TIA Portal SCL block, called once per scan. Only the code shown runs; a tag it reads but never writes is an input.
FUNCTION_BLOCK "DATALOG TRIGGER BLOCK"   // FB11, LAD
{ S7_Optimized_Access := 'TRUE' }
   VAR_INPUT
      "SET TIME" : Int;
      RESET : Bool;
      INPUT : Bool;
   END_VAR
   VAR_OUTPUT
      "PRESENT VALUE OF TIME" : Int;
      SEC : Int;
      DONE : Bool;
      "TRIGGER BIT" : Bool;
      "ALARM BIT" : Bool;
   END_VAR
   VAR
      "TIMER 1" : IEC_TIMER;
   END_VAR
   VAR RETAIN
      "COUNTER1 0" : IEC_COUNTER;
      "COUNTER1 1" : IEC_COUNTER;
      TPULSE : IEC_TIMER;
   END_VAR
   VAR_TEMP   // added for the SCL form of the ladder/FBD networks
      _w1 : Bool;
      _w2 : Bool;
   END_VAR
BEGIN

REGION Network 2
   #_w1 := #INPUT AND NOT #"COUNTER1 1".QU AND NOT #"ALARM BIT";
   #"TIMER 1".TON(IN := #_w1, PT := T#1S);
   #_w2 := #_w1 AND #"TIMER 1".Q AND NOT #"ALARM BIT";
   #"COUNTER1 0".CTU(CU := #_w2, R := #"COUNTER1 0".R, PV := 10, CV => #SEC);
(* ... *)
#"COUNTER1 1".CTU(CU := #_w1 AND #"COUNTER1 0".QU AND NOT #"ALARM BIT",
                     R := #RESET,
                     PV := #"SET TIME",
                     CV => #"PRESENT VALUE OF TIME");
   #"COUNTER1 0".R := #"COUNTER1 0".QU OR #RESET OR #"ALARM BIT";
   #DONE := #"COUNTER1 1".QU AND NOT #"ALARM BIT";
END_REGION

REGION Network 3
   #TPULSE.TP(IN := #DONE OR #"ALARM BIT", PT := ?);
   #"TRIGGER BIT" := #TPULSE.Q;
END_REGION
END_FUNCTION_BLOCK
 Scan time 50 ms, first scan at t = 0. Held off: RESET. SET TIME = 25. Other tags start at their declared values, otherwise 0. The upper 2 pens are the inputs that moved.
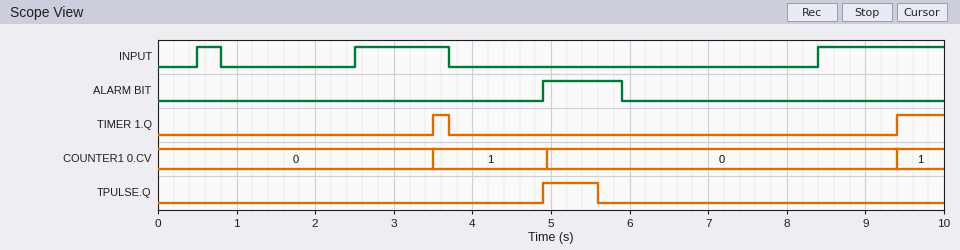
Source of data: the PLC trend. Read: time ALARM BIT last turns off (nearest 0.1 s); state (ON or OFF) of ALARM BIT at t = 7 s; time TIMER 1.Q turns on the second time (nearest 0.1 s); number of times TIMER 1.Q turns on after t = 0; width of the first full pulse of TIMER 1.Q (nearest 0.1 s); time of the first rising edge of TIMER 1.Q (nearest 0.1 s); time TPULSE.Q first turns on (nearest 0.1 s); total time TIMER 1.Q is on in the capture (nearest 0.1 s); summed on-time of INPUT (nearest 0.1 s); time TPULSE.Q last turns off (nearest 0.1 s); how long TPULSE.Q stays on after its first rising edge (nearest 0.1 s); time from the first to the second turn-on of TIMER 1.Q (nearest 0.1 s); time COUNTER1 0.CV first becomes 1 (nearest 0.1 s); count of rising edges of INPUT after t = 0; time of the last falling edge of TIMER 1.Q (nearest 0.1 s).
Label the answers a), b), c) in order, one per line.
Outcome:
a) 5.9 s
b) OFF
c) 9.4 s
d) 2
e) 0.2 s
f) 3.5 s
g) 4.9 s
h) 0.8 s
i) 3.1 s
j) 5.6 s
k) 0.7 s
l) 5.9 s
m) 3.5 s
n) 3
o) 3.7 s
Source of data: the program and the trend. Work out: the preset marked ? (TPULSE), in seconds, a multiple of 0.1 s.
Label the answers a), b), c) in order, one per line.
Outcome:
a) 0.7 s
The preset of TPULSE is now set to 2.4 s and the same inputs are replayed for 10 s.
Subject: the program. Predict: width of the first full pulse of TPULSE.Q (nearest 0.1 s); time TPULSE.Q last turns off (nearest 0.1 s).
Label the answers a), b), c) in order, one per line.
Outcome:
a) 2.4 s
b) 7.3 s
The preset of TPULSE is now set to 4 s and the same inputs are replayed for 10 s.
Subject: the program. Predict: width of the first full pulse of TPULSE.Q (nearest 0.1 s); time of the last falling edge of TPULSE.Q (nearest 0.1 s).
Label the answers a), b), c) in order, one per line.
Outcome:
a) 4.0 s
b) 8.9 s
